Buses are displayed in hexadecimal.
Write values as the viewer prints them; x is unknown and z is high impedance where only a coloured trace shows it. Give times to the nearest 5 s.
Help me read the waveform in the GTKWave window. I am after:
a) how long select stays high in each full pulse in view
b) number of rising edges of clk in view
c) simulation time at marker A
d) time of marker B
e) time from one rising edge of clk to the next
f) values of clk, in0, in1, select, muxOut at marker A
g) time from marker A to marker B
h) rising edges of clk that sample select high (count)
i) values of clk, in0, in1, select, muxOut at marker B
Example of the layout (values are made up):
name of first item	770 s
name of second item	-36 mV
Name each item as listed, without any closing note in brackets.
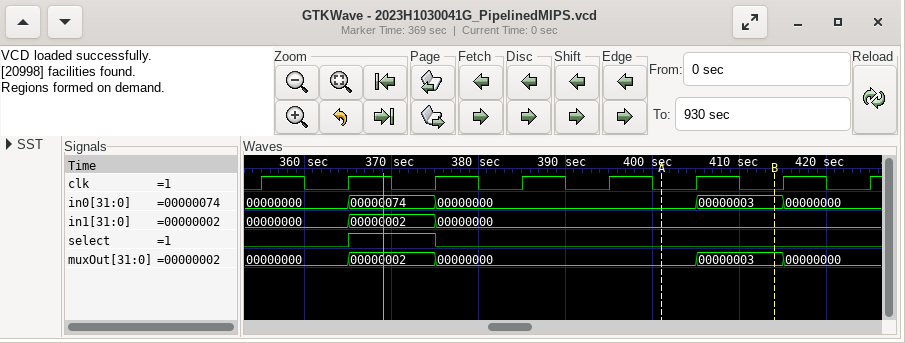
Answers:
how long select stays high in each full pulse in view	10 s
number of rising edges of clk in view	8
simulation time at marker A	400 s
time of marker B	415 s
time from one rising edge of clk to the next	10 s
values of clk, in0, in1, select, muxOut at marker A	clk=0, in0=00000000, in1=00000000, select=0, muxOut=00000000
time from marker A to marker B	15 s
rising edges of clk that sample select high	1
values of clk, in0, in1, select, muxOut at marker B	clk=0, in0=00000003, in1=00000000, select=0, muxOut=00000003
